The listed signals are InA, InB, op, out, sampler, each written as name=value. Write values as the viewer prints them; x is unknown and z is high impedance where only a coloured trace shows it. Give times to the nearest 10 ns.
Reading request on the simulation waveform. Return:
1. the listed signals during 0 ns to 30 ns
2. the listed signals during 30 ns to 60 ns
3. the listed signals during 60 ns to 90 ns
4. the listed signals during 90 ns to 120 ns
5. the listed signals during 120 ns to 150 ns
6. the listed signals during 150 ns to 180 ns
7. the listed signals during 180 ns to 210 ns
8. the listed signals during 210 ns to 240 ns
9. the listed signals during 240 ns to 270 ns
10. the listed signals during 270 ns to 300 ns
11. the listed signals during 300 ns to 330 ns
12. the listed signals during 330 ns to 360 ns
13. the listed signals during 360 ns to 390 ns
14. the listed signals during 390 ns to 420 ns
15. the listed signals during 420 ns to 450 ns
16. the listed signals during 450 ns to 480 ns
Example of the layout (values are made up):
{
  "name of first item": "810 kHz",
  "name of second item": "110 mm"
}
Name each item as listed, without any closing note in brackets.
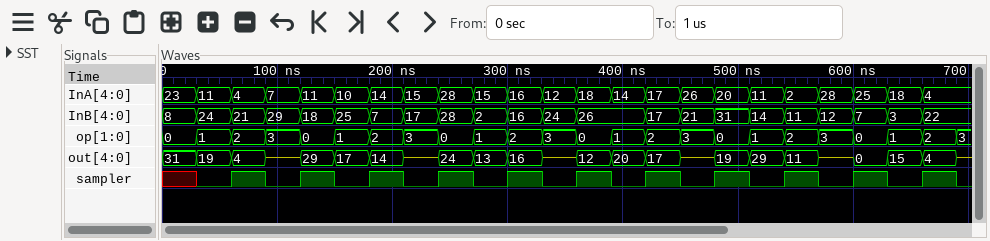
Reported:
{
  "the listed signals during 0 ns to 30 ns": "InA=23, InB=8, op=0, out=31, sampler=x",
  "the listed signals during 30 ns to 60 ns": "InA=11, InB=24, op=1, out=19, sampler=0",
  "the listed signals during 60 ns to 90 ns": "InA=4, InB=21, op=2, out=4, sampler=1",
  "the listed signals during 90 ns to 120 ns": "InA=7, InB=29, op=3, out=z, sampler=0",
  "the listed signals during 120 ns to 150 ns": "InA=11, InB=18, op=0, out=29, sampler=1",
  "the listed signals during 150 ns to 180 ns": "InA=10, InB=25, op=1, out=17, sampler=0",
  "the listed signals during 180 ns to 210 ns": "InA=14, InB=7, op=2, out=14, sampler=1",
  "the listed signals during 210 ns to 240 ns": "InA=15, InB=17, op=3, out=z, sampler=0",
  "the listed signals during 240 ns to 270 ns": "InA=28, InB=28, op=0, out=24, sampler=1",
  "the listed signals during 270 ns to 300 ns": "InA=15, InB=2, op=1, out=13, sampler=0",
  "the listed signals during 300 ns to 330 ns": "InA=16, InB=16, op=2, out=16, sampler=1",
  "the listed signals during 330 ns to 360 ns": "InA=12, InB=24, op=3, out=z, sampler=0",
  "the listed signals during 360 ns to 390 ns": "InA=18, InB=26, op=0, out=12, sampler=1",
  "the listed signals during 390 ns to 420 ns": "InA=14, InB=26, op=1, out=20, sampler=0",
  "the listed signals during 420 ns to 450 ns": "InA=17, InB=17, op=2, out=17, sampler=1",
  "the listed signals during 450 ns to 480 ns": "InA=26, InB=21, op=3, out=z, sampler=0"
}
